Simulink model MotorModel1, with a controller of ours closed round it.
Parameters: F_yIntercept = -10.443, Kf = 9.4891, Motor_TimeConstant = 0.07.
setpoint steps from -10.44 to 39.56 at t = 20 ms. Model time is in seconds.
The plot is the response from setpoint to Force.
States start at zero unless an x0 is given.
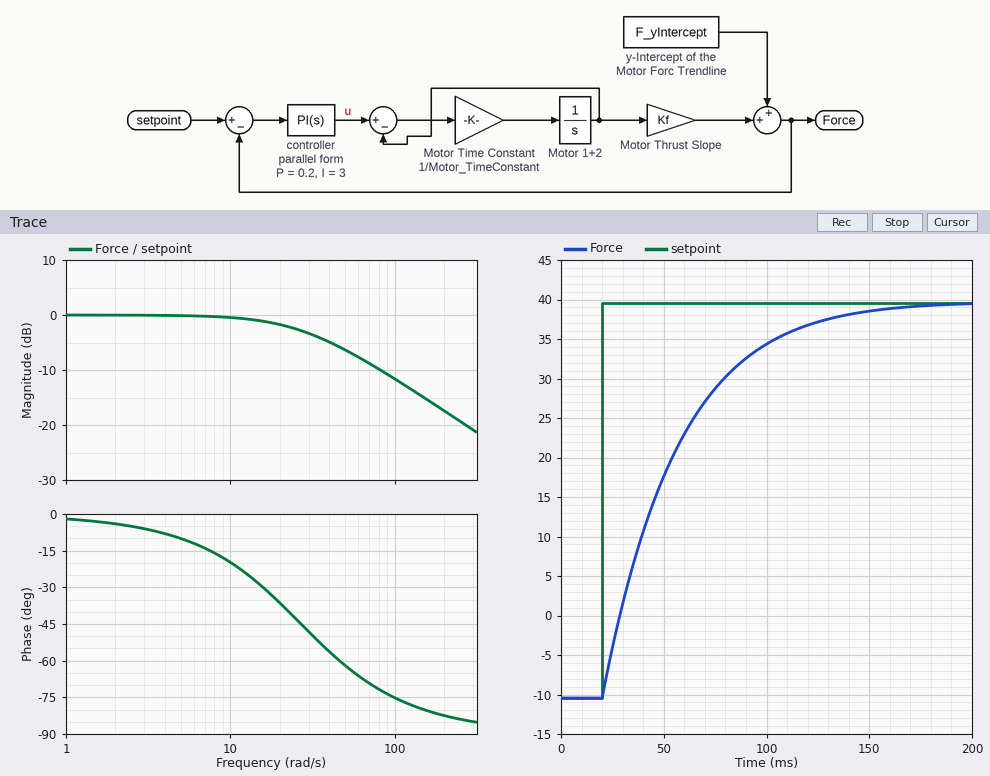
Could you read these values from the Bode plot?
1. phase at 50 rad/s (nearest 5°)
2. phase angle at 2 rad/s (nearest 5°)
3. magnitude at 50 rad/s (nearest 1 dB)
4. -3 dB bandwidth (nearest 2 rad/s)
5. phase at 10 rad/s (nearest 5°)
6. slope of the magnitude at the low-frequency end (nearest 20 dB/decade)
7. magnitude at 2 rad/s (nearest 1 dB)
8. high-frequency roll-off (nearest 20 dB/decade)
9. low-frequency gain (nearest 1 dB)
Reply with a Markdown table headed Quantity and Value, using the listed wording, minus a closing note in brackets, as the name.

| Quantity | Value |
|---|---|
| phase at 50 rad/s | -60° |
| phase angle at 2 rad/s | -5° |
| magnitude at 50 rad/s | -6 dB |
| -3 dB bandwidth | 28 rad/s |
| phase at 10 rad/s | -20° |
| slope of the magnitude at the low-frequency end | 0 dB/decade |
| magnitude at 2 rad/s | 0 dB |
| high-frequency roll-off | -20 dB/decade |
| low-frequency gain | 0 dB |
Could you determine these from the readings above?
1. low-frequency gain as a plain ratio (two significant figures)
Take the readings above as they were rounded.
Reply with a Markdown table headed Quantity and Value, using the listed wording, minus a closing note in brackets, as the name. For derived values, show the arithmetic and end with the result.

| Quantity | Value |
|---|---|
| low-frequency gain as a plain ratio | 10^(0 / 20) = 1.0 |
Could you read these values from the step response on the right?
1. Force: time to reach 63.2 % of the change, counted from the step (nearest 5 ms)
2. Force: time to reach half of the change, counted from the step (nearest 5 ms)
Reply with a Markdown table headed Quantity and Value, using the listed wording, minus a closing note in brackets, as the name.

| Quantity | Value |
|---|---|
| Force: time to reach 63.2 % of the change, counted from the step | 35 ms |
| Force: time to reach half of the change, counted from the step | 25 ms |
